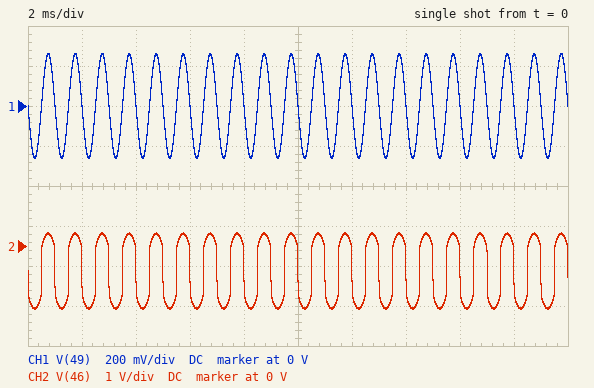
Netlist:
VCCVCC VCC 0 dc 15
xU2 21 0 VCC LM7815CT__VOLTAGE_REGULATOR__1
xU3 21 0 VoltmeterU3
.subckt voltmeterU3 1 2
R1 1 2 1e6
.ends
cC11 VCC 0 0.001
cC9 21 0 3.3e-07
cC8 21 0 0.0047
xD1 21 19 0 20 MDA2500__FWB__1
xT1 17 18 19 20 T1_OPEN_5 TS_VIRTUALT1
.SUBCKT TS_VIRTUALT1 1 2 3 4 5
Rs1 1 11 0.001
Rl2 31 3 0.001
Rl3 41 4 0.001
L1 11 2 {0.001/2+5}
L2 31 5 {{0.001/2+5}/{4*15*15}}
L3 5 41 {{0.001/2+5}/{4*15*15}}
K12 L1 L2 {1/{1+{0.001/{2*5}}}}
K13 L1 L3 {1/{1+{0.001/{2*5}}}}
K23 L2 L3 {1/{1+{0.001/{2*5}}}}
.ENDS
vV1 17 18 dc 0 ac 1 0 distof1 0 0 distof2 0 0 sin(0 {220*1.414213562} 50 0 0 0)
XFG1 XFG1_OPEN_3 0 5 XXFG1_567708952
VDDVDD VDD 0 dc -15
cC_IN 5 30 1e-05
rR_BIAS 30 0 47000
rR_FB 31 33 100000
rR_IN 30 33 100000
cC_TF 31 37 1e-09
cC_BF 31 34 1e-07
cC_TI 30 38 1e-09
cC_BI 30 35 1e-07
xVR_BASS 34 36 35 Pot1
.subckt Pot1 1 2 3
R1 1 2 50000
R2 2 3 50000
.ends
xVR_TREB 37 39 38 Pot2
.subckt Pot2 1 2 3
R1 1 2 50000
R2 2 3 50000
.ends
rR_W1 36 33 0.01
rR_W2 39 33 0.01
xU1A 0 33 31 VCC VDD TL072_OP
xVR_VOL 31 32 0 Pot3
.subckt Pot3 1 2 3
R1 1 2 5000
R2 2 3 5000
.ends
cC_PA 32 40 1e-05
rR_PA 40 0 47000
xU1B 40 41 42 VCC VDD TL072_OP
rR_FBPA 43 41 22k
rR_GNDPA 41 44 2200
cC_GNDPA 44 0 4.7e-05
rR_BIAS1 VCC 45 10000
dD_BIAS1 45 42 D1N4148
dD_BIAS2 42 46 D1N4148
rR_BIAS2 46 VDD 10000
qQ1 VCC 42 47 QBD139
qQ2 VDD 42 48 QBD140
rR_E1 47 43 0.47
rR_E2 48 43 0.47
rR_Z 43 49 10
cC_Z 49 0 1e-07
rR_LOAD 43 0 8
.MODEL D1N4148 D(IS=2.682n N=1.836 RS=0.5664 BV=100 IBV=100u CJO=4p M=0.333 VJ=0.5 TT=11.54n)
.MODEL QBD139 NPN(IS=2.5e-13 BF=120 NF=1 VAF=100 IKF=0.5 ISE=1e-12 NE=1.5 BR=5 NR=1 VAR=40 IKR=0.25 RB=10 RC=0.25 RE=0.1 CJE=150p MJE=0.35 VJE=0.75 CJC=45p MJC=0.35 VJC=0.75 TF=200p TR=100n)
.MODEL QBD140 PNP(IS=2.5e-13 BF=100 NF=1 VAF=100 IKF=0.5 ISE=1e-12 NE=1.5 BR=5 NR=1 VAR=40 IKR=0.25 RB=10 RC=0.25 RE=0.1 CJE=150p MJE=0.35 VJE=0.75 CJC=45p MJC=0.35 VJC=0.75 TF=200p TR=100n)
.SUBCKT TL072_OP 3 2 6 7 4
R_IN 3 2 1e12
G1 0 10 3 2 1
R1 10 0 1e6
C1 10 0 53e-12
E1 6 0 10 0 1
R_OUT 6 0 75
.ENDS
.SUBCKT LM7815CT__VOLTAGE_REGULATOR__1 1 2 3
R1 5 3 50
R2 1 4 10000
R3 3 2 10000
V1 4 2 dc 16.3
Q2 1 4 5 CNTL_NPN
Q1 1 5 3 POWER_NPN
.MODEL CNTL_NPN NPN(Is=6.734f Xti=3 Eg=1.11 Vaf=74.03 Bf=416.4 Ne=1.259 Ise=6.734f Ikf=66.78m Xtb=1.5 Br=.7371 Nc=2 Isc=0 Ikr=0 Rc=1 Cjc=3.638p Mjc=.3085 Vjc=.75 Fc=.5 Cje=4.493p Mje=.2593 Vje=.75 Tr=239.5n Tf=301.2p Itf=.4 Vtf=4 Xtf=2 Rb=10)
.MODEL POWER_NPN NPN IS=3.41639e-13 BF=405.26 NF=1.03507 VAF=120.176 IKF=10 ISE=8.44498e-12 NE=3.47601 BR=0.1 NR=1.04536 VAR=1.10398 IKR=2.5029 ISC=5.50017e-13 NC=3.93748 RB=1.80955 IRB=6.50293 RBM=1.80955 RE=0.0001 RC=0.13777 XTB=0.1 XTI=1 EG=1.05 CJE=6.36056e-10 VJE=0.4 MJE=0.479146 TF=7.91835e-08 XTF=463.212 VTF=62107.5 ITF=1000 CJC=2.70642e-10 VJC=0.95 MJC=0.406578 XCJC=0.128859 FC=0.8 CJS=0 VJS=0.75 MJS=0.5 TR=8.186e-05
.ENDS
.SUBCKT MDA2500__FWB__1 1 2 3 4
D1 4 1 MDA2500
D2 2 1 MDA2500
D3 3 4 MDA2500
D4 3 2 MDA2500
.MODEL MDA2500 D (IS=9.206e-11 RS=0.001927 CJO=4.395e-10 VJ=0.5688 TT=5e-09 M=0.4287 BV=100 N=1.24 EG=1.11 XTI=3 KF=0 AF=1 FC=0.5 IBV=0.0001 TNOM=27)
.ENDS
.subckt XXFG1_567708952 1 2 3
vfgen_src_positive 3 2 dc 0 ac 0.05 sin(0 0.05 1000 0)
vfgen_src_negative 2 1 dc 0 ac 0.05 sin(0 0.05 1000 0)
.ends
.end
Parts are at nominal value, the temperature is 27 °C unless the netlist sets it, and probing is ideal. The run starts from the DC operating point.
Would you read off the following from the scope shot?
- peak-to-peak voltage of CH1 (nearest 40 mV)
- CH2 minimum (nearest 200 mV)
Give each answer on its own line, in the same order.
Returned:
520 mV
-1.6 V
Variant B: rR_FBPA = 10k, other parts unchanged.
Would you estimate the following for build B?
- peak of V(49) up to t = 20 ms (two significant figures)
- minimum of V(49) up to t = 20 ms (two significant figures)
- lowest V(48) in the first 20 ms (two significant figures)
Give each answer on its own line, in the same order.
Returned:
130 mV
-130 mV
-140 mV
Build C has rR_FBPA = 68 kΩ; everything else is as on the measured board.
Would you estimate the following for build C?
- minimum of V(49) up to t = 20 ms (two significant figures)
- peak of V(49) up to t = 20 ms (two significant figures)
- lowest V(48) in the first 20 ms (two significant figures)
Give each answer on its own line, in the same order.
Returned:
-760 mV
760 mV
-800 mV
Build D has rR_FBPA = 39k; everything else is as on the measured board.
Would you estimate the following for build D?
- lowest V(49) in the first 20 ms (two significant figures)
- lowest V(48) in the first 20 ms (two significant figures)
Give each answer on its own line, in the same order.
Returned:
-440 mV
-470 mV
